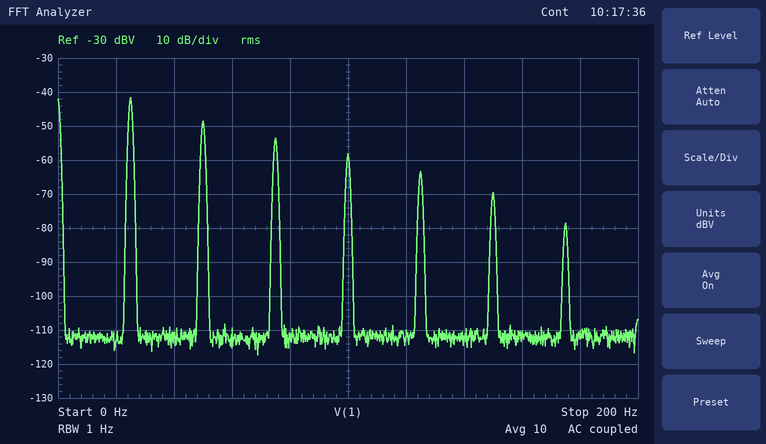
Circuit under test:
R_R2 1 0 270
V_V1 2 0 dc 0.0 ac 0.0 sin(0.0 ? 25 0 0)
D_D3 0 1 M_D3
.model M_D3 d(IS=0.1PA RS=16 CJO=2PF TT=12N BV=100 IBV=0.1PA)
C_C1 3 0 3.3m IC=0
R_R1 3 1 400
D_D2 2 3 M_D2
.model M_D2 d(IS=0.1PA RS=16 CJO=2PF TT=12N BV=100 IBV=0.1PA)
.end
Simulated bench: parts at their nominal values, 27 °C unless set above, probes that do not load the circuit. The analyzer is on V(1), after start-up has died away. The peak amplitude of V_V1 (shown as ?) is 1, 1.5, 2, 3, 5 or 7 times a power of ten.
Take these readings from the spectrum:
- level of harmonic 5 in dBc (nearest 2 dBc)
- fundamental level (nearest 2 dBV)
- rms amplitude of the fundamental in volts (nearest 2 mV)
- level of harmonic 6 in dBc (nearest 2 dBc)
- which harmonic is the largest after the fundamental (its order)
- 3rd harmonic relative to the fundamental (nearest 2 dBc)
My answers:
-22 dBc
-42 dBV
8 mV
-28 dBc
2
-12 dBc
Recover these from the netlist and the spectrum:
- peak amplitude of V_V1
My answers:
7 V
